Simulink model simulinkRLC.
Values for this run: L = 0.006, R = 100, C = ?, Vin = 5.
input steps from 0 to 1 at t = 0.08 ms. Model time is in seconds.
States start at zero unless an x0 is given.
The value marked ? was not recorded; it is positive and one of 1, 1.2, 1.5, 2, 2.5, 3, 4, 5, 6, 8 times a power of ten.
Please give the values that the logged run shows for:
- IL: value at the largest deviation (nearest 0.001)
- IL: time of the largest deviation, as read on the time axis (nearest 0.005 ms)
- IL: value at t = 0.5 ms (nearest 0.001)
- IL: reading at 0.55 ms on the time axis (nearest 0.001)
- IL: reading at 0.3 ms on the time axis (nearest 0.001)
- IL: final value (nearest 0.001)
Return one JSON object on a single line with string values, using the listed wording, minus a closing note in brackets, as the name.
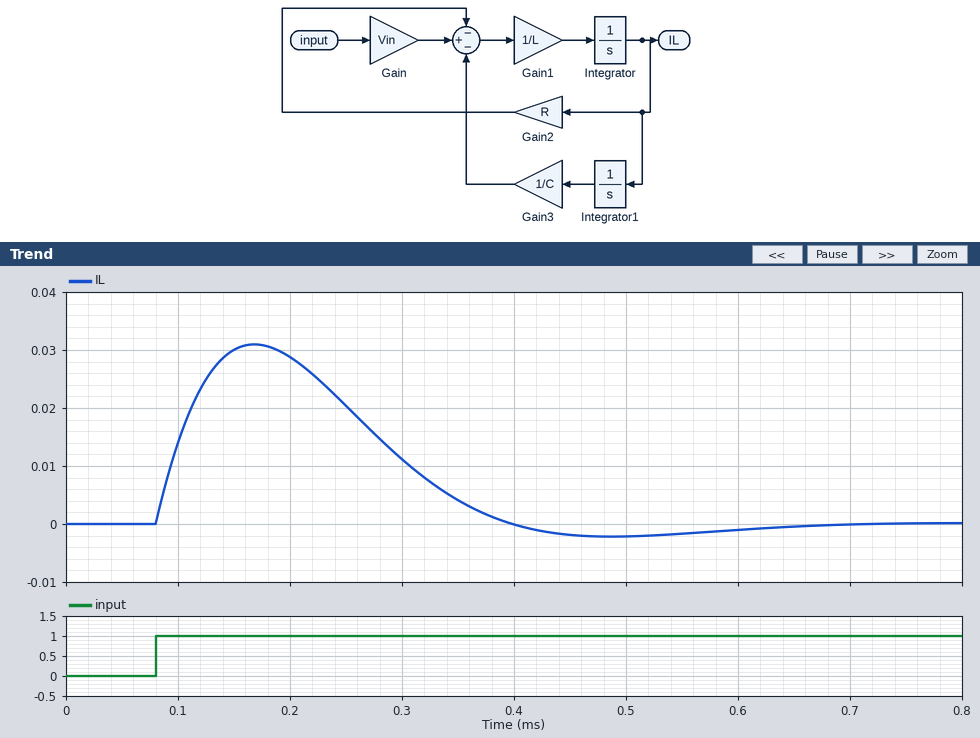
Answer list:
{"IL: value at the largest deviation": "0.031", "IL: time of the largest deviation, as read on the time axis": "0.170 ms", "IL: value at t = 0.5 ms": "-0.002", "IL: reading at 0.55 ms on the time axis": "-0.002", "IL: reading at 0.3 ms on the time axis": "0.011", "IL: final value": "0.000"}
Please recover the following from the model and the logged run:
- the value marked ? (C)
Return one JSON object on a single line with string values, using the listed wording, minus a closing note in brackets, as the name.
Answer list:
{"the value marked ?": "1e-06"}
